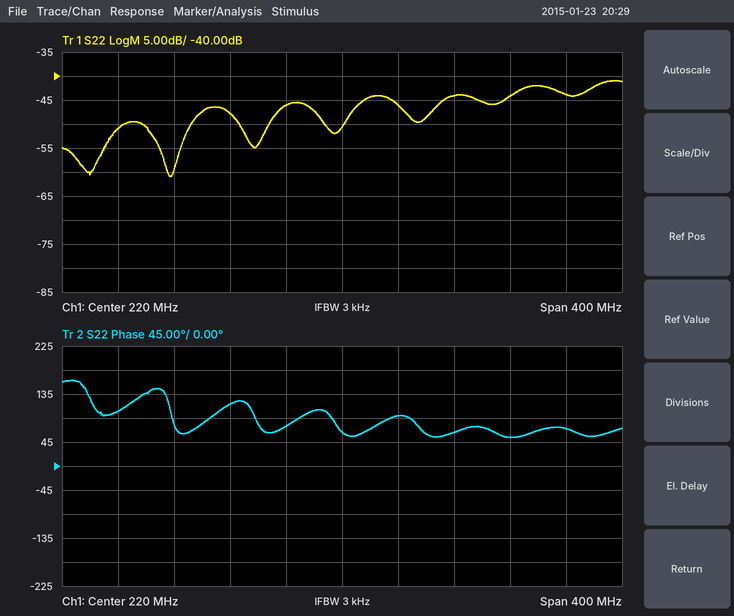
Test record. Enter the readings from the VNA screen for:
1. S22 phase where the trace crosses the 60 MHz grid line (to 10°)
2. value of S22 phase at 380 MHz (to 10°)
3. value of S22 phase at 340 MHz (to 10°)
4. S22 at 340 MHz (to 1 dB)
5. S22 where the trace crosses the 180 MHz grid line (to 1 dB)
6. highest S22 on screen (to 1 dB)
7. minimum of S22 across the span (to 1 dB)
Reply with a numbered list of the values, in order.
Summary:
1. 100°
2. 70°
3. 50°
4. -44 dB
5. -46 dB
6. -41 dB
7. -61 dB
